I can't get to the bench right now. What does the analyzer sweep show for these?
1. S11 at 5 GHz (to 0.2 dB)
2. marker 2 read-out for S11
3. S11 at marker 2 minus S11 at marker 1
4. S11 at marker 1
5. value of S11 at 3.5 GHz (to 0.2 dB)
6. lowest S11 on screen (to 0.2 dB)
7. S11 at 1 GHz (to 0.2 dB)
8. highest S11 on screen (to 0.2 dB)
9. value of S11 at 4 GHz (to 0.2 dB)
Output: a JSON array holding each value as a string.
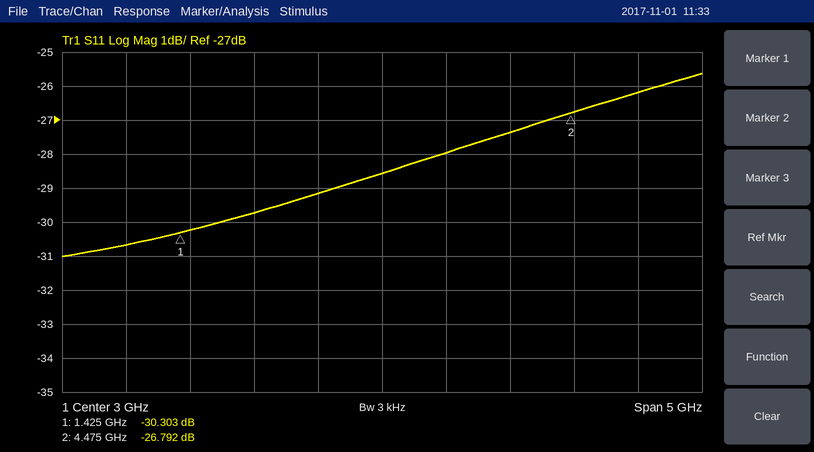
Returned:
["-26.2 dB", "-26.792 dB", "3.511 dB", "-30.303 dB", "-28.0 dB", "-31.0 dB", "-30.6 dB", "-25.6 dB", "-27.4 dB"]
